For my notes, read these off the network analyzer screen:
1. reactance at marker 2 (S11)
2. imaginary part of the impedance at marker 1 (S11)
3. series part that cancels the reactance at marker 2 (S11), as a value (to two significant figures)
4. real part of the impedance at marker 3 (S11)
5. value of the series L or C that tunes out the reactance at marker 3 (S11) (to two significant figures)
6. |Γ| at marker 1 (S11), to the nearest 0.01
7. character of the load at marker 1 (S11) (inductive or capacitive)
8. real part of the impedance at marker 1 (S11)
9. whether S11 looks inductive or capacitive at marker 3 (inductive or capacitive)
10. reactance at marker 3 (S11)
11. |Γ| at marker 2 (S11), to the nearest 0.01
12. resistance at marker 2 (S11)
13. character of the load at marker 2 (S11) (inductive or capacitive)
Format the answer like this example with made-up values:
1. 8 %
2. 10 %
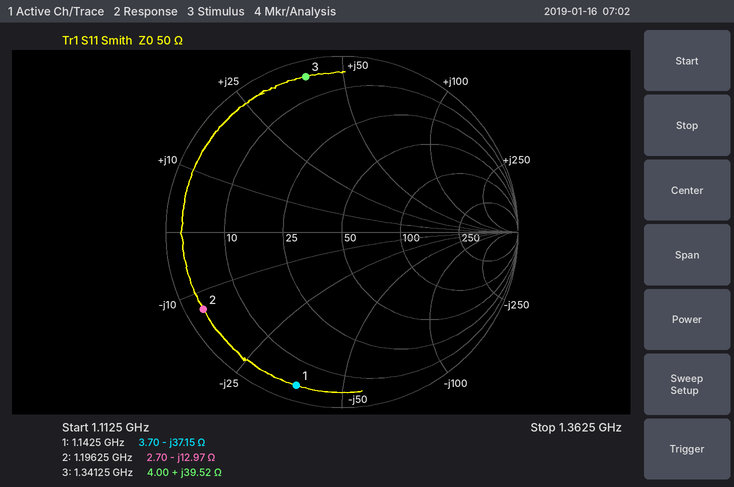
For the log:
1. -12.97 Ω
2. -37.15 Ω
3. 1.7 nH
4. 4.00 Ω
5. 3.0 pF
6. 0.91
7. capacitive
8. 3.70 Ω
9. inductive
10. +39.52 Ω
11. 0.90
12. 2.70 Ω
13. capacitive
